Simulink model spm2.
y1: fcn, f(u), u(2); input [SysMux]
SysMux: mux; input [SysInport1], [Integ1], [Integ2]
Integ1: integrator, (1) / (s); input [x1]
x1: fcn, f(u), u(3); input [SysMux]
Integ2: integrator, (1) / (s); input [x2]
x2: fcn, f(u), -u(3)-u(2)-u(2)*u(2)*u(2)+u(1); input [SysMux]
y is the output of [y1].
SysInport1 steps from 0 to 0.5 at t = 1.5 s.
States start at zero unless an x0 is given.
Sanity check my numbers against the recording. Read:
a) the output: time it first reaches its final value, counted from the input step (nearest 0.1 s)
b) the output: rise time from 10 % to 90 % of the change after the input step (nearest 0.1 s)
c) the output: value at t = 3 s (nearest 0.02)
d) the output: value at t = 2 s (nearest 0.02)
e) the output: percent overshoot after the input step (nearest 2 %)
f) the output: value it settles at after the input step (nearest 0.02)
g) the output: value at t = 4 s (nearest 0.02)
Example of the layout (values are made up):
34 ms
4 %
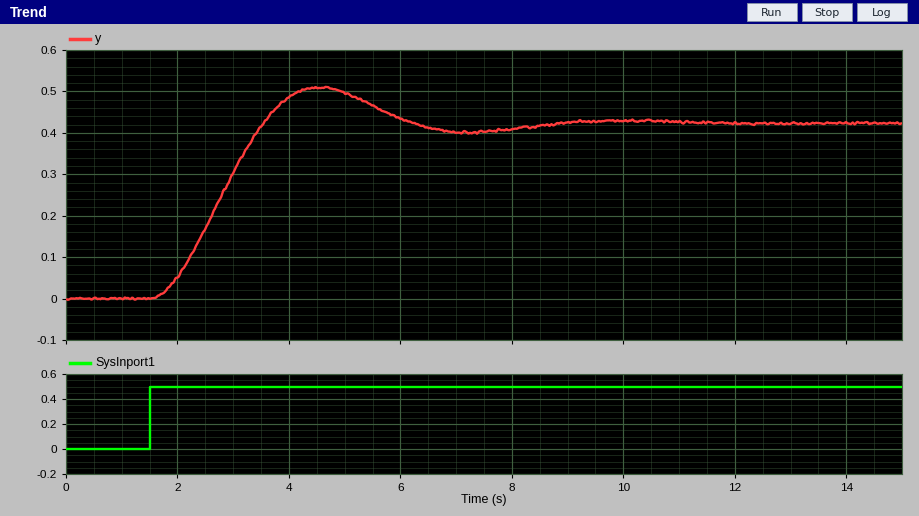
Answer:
2.0 s
1.4 s
0.30
0.06
20 %
0.42
0.48
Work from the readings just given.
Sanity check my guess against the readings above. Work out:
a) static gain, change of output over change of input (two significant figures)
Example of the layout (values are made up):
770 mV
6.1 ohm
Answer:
0.84
